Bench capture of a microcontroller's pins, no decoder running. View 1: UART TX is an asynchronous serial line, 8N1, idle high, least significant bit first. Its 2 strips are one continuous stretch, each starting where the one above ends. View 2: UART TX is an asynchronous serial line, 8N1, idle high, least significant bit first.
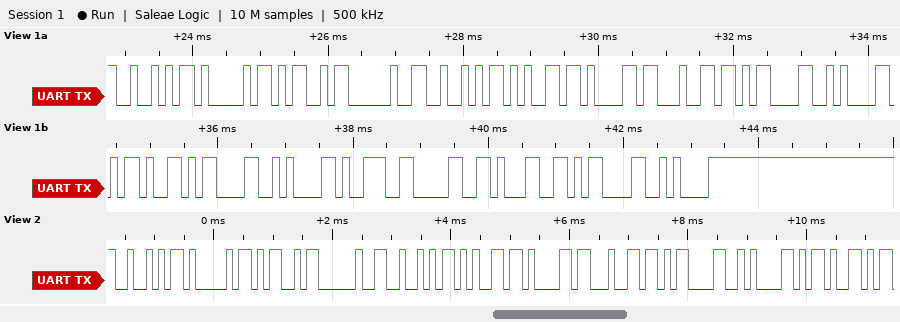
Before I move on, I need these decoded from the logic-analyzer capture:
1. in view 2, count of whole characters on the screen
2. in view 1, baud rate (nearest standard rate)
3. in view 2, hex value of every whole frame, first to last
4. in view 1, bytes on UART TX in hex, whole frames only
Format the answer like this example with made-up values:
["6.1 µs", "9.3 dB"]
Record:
["11", "9600 baud", "52 41 4D 20 52 65 61 64 0D 0A 2D", "52 41 4D 20 52 65 61 64 0D 0A 2D 0D 0A 39 30 31 0D 0A"]
